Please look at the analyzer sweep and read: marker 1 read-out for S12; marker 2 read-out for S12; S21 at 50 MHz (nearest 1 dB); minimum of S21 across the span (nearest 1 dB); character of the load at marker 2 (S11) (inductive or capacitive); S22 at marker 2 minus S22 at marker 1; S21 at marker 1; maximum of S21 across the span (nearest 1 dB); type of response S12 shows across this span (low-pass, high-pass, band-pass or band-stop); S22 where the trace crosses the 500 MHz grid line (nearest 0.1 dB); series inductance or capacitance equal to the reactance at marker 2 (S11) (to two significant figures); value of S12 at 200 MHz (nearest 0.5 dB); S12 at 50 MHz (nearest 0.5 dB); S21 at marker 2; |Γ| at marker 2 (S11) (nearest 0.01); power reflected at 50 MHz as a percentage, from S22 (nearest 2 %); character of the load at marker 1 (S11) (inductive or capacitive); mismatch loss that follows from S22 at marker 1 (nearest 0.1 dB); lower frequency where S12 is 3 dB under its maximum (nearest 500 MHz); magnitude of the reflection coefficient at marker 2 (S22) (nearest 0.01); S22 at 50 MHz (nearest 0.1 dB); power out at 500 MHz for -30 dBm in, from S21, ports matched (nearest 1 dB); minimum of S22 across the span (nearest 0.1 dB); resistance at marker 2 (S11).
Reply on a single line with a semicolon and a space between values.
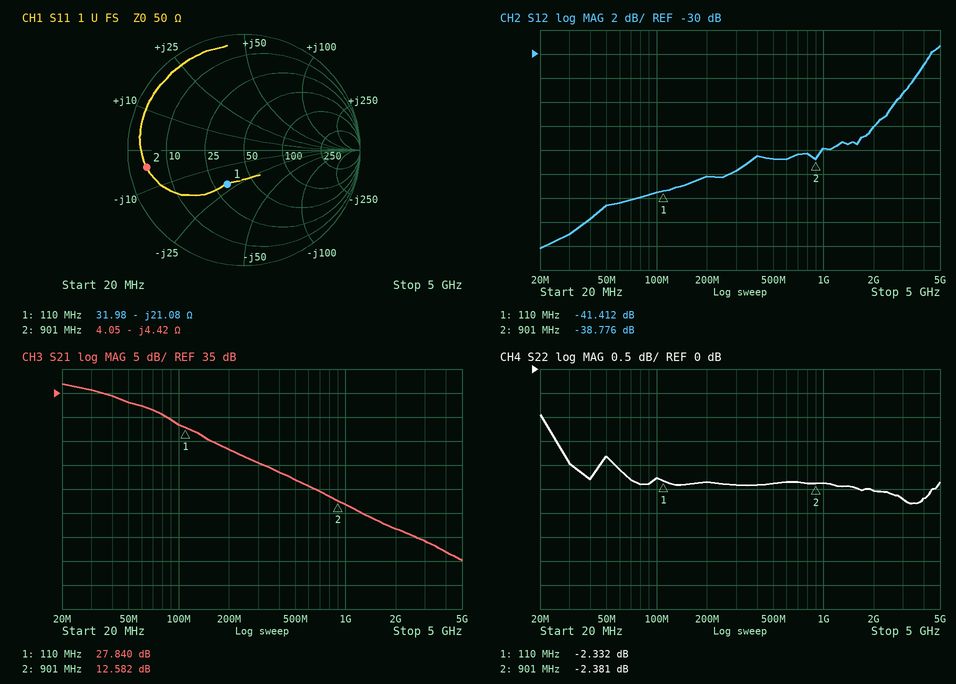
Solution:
-41.412 dB; -38.776 dB; 33 dB; 0 dB; capacitive; -0.049 dB; 27.840 dB; 37 dB; high-pass; -2.4 dB; 40 pF; -40.0 dB; -42.5 dB; 12.582 dB; 0.85; 66 %; capacitive; 3.8 dB; 3.5 GHz; 0.76; -1.8 dB; -13 dBm; -2.8 dB; 4.05 Ω
